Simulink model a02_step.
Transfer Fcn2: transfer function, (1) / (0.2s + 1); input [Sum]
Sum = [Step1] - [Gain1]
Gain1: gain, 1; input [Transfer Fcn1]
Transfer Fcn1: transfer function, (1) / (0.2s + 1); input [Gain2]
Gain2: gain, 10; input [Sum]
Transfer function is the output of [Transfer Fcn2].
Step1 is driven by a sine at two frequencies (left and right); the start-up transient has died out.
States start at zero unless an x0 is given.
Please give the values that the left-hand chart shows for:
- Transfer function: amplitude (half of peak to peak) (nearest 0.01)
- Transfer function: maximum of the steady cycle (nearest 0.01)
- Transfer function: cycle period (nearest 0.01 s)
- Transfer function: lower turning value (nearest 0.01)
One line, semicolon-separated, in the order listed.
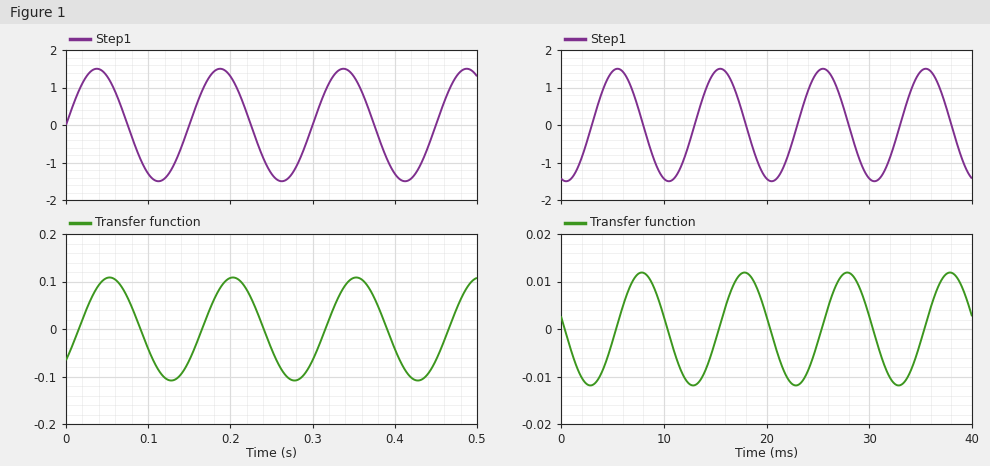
0.11; 0.11; 0.15 s; -0.11
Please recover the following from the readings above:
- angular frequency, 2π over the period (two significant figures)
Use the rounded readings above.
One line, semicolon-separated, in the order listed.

42 rad/s
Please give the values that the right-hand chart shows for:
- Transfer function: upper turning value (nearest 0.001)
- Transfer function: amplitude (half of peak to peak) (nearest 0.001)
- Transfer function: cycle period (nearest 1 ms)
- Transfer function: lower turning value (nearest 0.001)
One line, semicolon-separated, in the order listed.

0.012; 0.012; 10 ms; -0.012
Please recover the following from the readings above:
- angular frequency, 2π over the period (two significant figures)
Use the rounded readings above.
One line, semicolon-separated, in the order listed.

0.63 rad/ms
